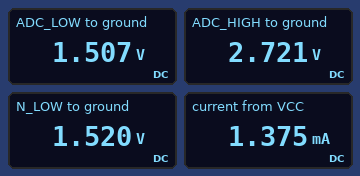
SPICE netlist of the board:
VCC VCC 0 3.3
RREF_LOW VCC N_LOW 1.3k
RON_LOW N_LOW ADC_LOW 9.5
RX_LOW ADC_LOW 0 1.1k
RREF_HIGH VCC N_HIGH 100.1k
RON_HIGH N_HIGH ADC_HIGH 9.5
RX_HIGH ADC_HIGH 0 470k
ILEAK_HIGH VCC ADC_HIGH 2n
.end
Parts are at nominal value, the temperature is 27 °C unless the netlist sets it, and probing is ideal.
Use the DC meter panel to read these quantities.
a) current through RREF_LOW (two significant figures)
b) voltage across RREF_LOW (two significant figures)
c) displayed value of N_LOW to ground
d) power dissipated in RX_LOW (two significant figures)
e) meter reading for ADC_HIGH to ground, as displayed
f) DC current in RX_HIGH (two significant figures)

1.4 mA
1.8 V
1.520 V
2.1 mW
2.721 V
5.8 µA
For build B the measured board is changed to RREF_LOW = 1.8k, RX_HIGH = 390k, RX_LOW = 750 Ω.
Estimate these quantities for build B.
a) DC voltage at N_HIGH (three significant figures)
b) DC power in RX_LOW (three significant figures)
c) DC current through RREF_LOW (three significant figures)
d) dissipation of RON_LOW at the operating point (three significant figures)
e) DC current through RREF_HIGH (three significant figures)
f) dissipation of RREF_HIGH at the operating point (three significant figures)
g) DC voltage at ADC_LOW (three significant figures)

2.63 V
1.25 mW
1.29 mA
15.8 µW
6.73 µA
4.54 µW
967 mV
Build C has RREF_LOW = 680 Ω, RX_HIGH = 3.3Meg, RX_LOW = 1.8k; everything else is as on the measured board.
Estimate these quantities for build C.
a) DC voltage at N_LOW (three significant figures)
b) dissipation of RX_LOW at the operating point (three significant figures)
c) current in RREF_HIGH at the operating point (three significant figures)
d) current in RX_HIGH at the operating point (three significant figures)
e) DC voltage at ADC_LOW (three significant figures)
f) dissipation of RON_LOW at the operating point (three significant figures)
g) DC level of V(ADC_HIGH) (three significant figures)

2.40 V
3.16 mW
969 nA
971 nA
2.39 V
16.7 µW
3.20 V
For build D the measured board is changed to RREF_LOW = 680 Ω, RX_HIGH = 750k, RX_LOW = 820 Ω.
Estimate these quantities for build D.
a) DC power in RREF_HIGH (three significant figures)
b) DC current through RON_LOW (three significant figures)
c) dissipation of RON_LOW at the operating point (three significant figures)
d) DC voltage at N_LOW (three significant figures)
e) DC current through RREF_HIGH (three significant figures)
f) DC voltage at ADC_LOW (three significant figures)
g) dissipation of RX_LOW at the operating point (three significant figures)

1.51 µW
2.19 mA
45.4 µW
1.81 V
3.88 µA
1.79 V
3.92 mW
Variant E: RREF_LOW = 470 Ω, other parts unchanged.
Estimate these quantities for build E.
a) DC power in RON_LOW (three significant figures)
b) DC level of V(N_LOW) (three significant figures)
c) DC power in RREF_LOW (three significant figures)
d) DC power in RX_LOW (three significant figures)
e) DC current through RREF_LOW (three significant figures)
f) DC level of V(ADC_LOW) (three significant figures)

41.5 µW
2.32 V
2.05 mW
4.80 mW
2.09 mA
2.30 V
